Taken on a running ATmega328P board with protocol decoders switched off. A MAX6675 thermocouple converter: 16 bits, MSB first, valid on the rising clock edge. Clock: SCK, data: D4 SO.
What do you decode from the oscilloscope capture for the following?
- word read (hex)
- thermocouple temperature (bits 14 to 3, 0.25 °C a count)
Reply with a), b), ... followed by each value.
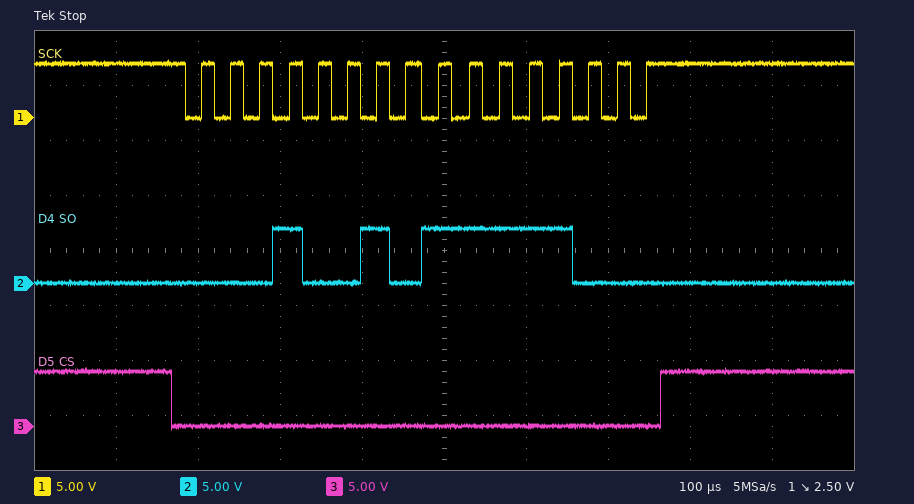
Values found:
a) 0x12F8
b) 151.75 °C
